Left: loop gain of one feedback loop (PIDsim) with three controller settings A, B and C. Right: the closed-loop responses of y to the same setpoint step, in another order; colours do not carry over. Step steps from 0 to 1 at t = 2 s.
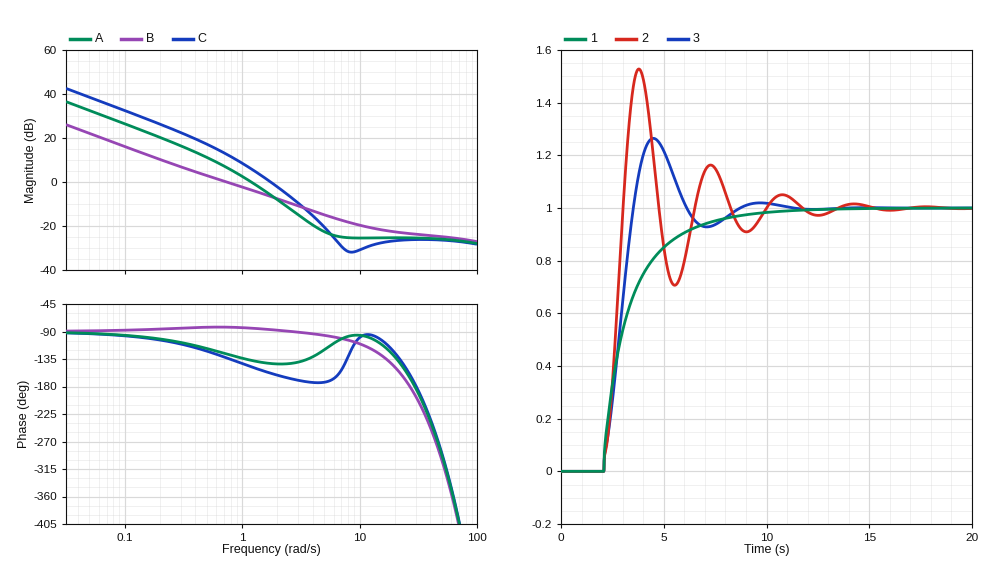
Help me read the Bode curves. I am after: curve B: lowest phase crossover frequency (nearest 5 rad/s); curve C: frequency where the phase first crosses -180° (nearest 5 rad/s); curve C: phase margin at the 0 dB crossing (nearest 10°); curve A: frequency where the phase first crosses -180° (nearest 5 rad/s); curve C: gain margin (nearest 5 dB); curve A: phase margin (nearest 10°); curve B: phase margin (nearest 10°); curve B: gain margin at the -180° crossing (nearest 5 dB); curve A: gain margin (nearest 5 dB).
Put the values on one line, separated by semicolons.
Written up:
25 rad/s; 30 rad/s; 20°; 30 rad/s; 25 dB; 40°; 100°; 25 dB; 25 dB
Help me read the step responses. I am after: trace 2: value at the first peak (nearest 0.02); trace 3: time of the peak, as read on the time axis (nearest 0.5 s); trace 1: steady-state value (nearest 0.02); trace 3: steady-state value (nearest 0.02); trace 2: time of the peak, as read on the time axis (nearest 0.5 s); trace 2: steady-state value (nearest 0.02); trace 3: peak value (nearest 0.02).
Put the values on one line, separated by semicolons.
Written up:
1.52; 4.5 s; 1.00; 1.00; 4.0 s; 1.00; 1.26
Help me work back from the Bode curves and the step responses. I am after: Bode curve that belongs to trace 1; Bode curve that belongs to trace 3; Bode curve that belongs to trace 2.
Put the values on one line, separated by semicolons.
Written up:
B; A; C
